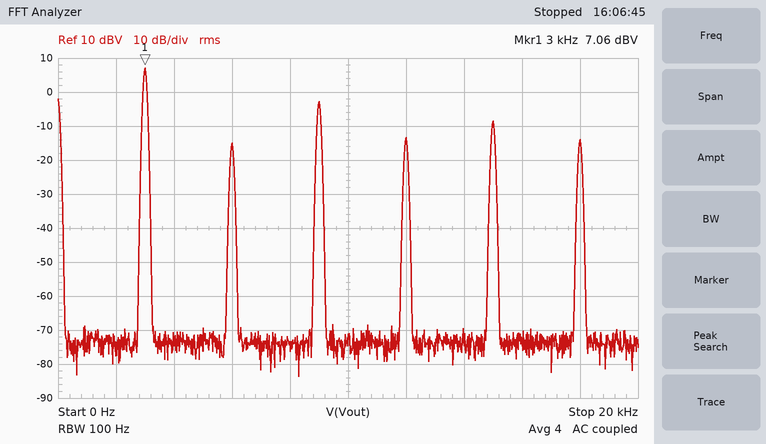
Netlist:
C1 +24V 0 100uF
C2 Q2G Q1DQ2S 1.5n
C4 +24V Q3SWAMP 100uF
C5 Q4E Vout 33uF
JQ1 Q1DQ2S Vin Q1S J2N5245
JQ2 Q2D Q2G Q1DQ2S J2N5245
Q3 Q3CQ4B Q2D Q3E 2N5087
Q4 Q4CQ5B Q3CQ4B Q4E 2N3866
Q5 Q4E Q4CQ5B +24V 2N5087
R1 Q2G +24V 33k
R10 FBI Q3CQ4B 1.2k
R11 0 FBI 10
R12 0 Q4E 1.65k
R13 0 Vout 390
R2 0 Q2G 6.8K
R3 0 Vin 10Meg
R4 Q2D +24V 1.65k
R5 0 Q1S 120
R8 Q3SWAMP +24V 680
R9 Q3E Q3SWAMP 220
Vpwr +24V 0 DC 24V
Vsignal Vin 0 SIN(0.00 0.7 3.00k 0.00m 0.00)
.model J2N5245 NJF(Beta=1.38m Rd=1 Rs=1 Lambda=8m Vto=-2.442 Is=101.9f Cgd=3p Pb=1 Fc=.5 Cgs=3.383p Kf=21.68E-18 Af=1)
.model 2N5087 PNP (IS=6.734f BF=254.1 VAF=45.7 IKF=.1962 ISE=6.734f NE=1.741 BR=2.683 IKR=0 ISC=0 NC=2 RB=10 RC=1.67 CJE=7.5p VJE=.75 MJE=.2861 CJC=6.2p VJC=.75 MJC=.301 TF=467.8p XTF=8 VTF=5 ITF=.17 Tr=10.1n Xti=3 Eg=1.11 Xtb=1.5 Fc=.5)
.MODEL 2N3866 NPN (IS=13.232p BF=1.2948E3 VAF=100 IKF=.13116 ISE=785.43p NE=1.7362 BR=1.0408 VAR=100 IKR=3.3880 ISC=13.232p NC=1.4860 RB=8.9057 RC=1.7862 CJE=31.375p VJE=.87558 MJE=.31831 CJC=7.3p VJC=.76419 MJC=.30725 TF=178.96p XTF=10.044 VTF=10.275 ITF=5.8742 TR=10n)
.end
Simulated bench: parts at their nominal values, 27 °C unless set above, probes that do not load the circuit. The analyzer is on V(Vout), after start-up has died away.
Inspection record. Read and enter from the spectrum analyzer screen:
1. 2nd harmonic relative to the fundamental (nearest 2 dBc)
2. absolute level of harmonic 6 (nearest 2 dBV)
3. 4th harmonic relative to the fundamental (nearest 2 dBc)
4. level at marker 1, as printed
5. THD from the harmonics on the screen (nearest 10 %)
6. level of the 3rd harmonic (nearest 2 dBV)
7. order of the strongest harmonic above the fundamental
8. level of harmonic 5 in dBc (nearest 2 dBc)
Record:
-22 dBc
-14 dBV
-20 dBc
7.06 dBV
40 %
-2 dBV
3
-16 dBc
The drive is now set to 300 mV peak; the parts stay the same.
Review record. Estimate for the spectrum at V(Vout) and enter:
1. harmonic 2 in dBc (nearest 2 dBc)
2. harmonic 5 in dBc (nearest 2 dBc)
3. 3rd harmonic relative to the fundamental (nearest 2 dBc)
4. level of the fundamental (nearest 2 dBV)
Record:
-10 dBc
-40 dBc
-16 dBc
8 dBV
